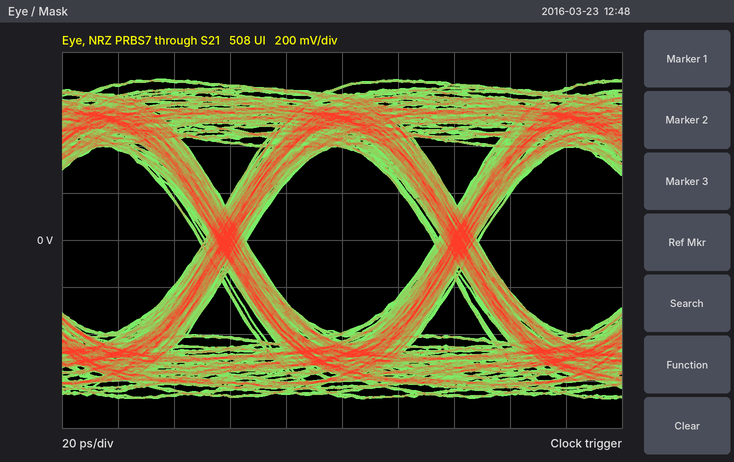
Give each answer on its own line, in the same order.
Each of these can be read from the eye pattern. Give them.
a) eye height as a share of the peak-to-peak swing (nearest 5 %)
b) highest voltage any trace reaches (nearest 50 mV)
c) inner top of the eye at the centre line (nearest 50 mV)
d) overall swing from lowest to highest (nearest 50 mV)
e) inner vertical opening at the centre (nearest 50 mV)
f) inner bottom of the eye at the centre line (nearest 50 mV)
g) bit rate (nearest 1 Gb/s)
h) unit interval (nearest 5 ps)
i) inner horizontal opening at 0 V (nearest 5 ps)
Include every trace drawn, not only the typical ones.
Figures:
60 %
700 mV
400 mV
1.35 V
800 mV
-400 mV
12 Gb/s
85 ps
65 ps
